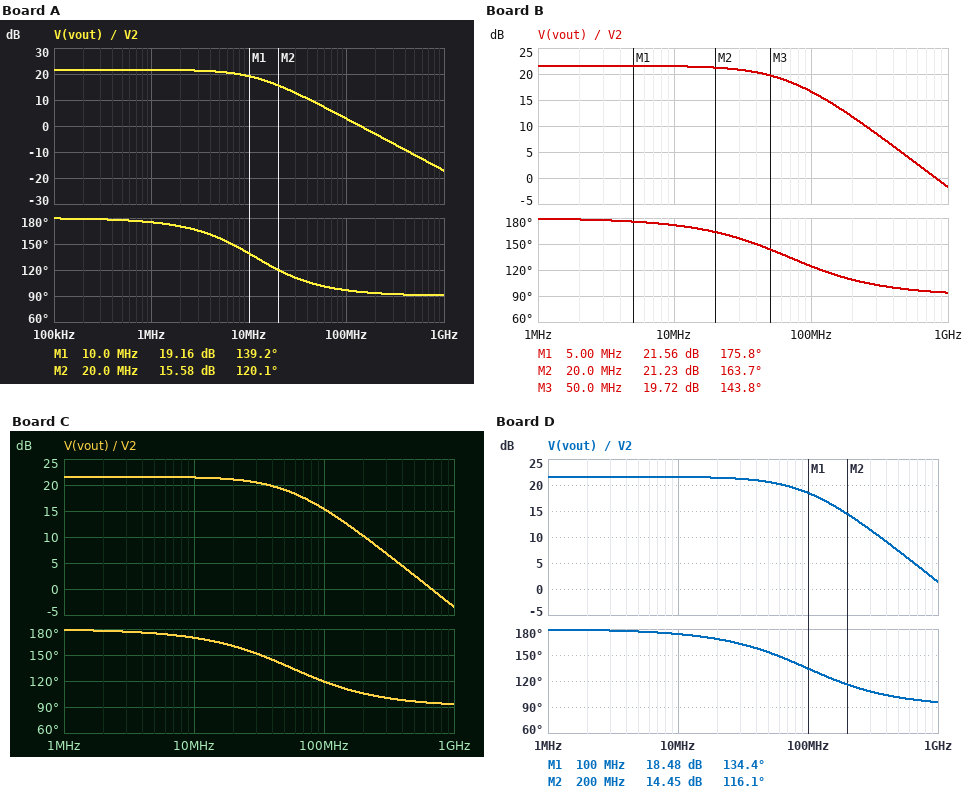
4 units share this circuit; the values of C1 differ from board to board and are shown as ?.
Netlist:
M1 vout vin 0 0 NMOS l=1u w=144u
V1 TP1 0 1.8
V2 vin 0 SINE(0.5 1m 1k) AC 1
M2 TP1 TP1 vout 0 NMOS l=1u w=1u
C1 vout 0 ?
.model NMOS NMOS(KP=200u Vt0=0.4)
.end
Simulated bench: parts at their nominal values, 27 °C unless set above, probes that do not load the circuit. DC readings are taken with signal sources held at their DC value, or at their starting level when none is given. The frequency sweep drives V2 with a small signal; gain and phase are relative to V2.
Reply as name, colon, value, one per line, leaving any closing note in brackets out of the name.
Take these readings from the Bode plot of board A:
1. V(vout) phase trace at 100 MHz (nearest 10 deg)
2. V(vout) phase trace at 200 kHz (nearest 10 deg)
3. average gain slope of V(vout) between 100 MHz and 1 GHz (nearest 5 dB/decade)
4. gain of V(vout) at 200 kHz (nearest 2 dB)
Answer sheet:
V(vout) phase trace at 100 MHz: 100 deg
V(vout) phase trace at 200 kHz: 180 deg
average gain slope of V(vout) between 100 MHz and 1 GHz: -20 dB/decade
gain of V(vout) at 200 kHz: 22 dB
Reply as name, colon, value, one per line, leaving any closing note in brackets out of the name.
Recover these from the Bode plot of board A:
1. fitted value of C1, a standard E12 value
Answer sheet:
fitted value of C1, a standard E12 value: 3.3 pF
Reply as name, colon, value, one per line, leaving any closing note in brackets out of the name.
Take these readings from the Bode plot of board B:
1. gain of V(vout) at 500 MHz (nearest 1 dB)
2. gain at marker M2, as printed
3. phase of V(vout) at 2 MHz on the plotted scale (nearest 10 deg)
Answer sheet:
gain of V(vout) at 500 MHz: 4 dB
gain at marker M2, as printed: 21.23 dB
phase of V(vout) at 2 MHz on the plotted scale: 180 deg
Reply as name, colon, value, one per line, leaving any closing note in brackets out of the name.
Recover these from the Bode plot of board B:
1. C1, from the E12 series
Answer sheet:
C1, from the E12 series: 560 fF
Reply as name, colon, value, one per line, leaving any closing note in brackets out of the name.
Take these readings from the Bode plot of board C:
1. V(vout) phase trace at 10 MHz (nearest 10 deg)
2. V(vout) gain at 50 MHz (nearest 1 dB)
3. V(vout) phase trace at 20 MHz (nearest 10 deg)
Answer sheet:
V(vout) phase trace at 10 MHz: 170 deg
V(vout) gain at 50 MHz: 19 dB
V(vout) phase trace at 20 MHz: 160 deg
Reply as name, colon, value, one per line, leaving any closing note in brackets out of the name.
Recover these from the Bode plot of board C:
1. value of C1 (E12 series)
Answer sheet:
value of C1: 680 fF
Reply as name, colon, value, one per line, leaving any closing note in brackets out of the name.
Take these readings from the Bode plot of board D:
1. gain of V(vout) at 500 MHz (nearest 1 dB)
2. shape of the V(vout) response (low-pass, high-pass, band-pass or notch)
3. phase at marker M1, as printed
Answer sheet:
gain of V(vout) at 500 MHz: 7 dB
shape of the V(vout) response: low-pass
phase at marker M1, as printed: 134.4 deg
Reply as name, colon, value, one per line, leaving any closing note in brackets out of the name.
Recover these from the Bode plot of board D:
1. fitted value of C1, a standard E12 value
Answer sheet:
fitted value of C1, a standard E12 value: 390 fF
